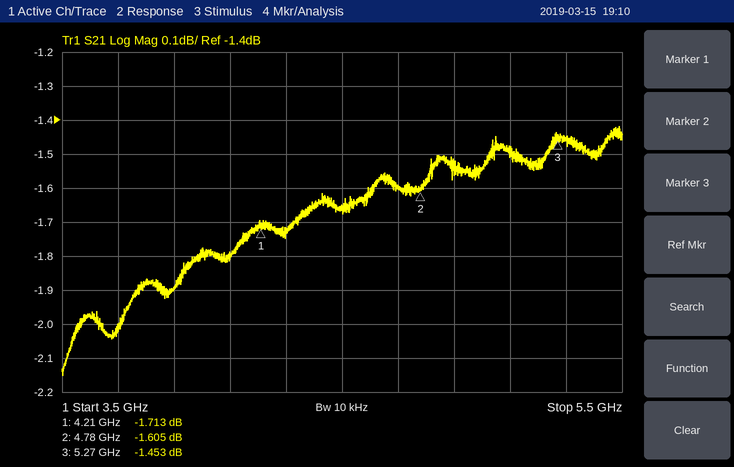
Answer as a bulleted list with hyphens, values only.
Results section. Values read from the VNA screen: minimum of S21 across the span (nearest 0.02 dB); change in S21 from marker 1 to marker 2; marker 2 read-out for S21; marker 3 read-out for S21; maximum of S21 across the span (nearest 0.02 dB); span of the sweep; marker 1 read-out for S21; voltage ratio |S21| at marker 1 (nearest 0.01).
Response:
- -2.16 dB
- 0.108 dB
- -1.605 dB
- -1.453 dB
- -1.42 dB
- 2 GHz
- -1.713 dB
- 0.82
